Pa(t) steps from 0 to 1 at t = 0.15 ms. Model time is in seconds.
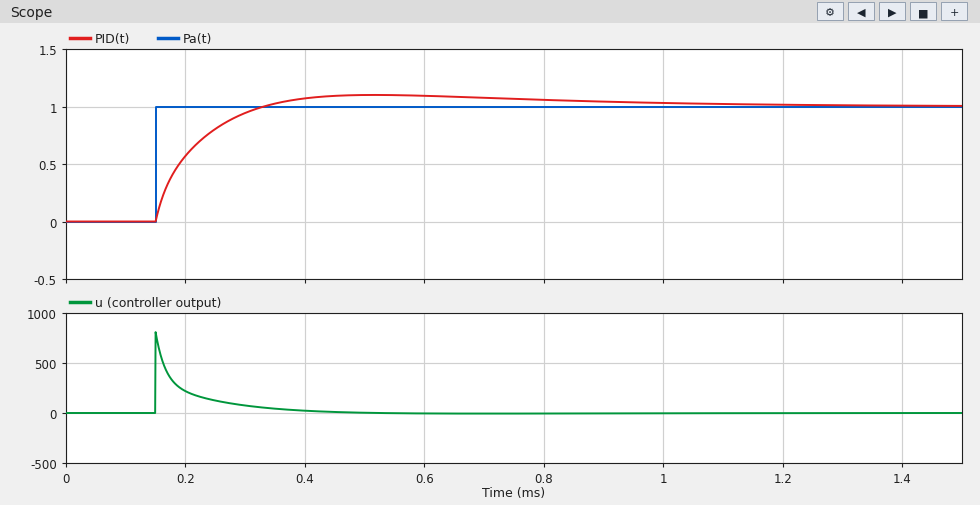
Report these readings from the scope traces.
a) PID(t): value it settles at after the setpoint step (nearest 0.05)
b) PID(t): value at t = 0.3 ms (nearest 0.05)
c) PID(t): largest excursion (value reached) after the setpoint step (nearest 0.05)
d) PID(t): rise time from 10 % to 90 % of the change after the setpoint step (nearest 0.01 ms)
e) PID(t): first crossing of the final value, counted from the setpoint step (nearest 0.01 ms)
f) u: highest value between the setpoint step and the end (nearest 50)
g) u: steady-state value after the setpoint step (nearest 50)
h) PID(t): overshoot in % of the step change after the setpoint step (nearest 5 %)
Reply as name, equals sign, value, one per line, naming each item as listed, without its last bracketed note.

PID(t): value it settles at after the setpoint step = 1.00
PID(t): value at t = 0.3 ms = 0.95
PID(t): largest excursion (value reached) after the setpoint step = 1.10
PID(t): rise time from 10 % to 90 % of the change after the setpoint step = 0.13 ms
PID(t): first crossing of the final value, counted from the setpoint step = 0.18 ms
u: highest value between the setpoint step and the end = 800
u: steady-state value after the setpoint step = 0
PID(t): overshoot in % of the step change after the setpoint step = 10 %
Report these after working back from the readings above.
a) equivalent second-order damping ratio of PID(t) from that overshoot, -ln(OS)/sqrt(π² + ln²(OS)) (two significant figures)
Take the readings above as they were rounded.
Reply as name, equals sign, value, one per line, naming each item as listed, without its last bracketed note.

equivalent second-order damping ratio of PID(t) from that overshoot, -ln(OS)/sqrt(π² + ln²(OS)) = 0.59
